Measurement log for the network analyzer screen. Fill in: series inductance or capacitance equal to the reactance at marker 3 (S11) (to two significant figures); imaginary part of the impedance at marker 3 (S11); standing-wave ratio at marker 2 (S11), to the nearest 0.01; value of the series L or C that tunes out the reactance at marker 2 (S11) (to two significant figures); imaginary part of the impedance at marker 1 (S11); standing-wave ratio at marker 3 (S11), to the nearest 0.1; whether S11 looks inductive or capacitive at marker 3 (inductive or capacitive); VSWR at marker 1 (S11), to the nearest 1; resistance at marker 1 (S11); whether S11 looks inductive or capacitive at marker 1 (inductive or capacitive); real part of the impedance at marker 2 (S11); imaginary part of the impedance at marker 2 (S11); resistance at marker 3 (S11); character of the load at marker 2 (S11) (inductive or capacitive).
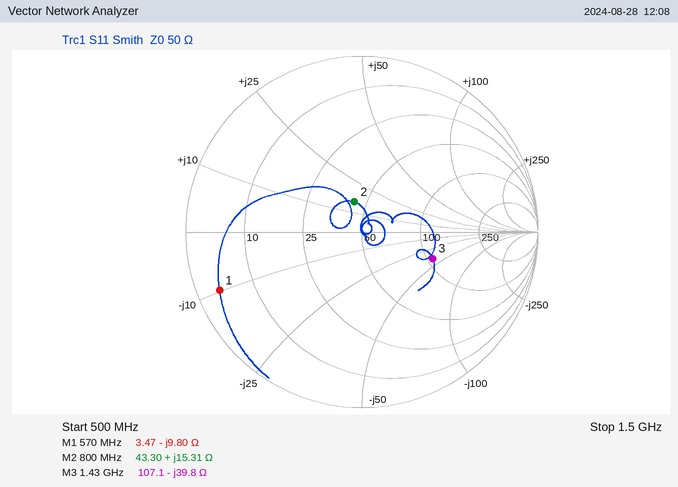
2.8 pF
-39.8 Ω
1.43
13 pF
-9.80 Ω
2.5
capacitive
15
3.47 Ω
capacitive
43.30 Ω
+15.31 Ω
107.1 Ω
inductive
